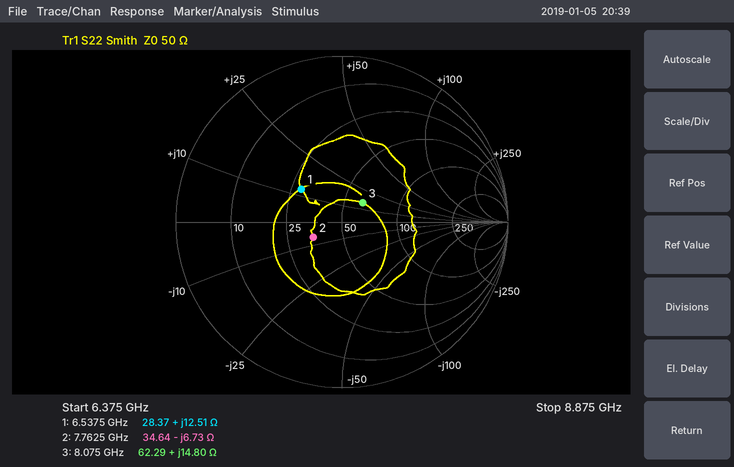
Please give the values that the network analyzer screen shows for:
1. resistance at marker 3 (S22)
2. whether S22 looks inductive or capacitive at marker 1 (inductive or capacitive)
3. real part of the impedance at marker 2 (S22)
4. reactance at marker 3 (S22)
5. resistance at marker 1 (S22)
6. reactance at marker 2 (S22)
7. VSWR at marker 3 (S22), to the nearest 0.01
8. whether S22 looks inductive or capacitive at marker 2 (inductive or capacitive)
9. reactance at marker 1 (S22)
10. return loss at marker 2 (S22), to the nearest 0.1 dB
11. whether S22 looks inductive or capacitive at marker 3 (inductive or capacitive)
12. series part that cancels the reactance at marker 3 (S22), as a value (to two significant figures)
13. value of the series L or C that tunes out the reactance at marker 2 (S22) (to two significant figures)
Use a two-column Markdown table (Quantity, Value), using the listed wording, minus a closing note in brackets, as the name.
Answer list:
| Quantity | Value |
|---|---|
| resistance at marker 3 | 62.29 Ω |
| whether S22 looks inductive or capacitive at marker 1 | inductive |
| real part of the impedance at marker 2 | 34.64 Ω |
| reactance at marker 3 | +14.80 Ω |
| resistance at marker 1 | 28.37 Ω |
| reactance at marker 2 | -6.73 Ω |
| VSWR at marker 3 (S22), to the nearest 0.01 | 1.41 |
| whether S22 looks inductive or capacitive at marker 2 | capacitive |
| reactance at marker 1 | +12.51 Ω |
| return loss at marker 2 (S22), to the nearest 0.1 dB | 14.1 dB |
| whether S22 looks inductive or capacitive at marker 3 | inductive |
| series part that cancels the reactance at marker 3 (S22), as a value | 1.3 pF |
| value of the series L or C that tunes out the reactance at marker 2 (S22) | 140 pH |
